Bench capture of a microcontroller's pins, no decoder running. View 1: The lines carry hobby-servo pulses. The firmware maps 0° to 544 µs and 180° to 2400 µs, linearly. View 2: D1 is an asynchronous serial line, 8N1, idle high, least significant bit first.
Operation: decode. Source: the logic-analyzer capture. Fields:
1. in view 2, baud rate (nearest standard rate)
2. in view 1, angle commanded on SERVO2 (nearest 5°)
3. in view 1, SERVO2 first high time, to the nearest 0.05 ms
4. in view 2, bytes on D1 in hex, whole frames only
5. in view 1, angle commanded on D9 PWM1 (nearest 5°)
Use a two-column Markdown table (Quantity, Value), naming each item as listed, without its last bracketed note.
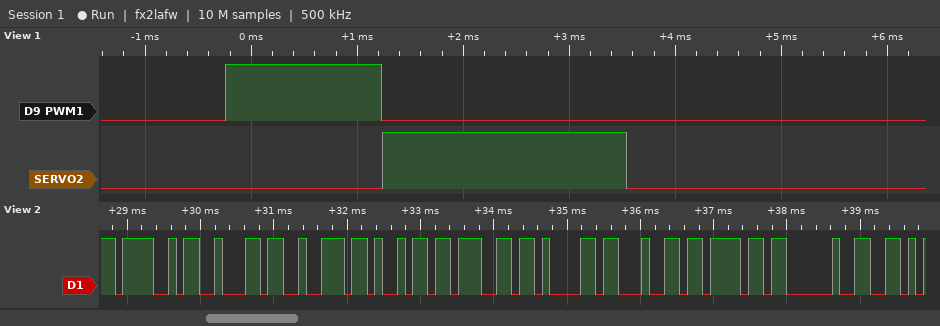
| Quantity | Value |
|---|---|
| in view 2, baud rate | 9600 baud |
| in view 1, angle commanded on SERVO2 | 170° |
| in view 1, SERVO2 first high time, to the nearest 0.05 ms | 2.30 ms |
| in view 2, bytes on D1 in hex, whole frames only | 0x4F 0x62 0x72 0x69 0x67 0x61 0x64 0x6F 0x20 |
| in view 1, angle commanded on D9 PWM1 | 90° |
